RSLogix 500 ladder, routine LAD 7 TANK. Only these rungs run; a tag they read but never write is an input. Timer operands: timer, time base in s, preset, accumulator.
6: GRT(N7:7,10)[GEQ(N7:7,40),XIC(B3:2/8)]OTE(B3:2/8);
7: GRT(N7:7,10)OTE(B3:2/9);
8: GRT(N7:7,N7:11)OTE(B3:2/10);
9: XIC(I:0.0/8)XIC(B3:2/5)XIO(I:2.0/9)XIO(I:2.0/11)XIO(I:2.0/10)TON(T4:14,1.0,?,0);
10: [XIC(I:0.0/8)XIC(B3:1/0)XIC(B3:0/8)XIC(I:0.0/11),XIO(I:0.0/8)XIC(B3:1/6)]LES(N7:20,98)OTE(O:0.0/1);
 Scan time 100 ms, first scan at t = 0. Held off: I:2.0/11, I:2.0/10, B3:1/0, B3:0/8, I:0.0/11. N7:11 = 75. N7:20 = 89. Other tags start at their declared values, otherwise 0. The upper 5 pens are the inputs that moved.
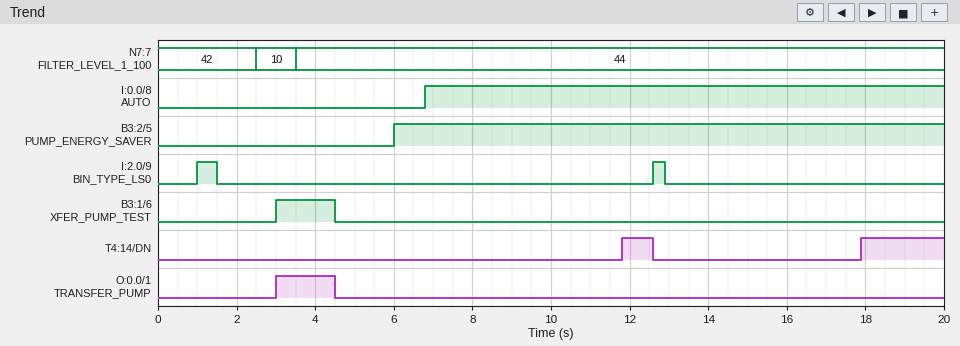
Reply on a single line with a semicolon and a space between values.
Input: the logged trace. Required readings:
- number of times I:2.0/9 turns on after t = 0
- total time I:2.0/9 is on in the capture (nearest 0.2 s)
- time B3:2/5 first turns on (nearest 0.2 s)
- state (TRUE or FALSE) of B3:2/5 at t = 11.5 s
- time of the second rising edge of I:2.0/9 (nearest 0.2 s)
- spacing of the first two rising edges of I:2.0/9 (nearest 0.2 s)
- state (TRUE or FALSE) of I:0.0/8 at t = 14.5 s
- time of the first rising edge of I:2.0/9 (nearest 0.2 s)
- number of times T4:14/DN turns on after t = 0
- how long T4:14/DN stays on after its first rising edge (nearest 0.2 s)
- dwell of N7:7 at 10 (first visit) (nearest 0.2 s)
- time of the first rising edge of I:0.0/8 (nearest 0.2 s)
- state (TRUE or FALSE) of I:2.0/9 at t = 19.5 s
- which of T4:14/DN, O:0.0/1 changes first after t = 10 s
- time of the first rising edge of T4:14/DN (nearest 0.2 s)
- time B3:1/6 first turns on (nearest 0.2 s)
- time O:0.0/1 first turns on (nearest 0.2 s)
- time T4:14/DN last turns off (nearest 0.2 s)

2; 0.8 s; 6.0 s; TRUE; 12.6 s; 11.6 s; TRUE; 1.0 s; 2; 0.8 s; 1.0 s; 6.8 s; FALSE; T4:14/DN; 11.8 s; 3.0 s; 3.0 s; 12.6 s
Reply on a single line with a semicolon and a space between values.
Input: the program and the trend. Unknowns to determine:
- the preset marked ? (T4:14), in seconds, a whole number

5 s
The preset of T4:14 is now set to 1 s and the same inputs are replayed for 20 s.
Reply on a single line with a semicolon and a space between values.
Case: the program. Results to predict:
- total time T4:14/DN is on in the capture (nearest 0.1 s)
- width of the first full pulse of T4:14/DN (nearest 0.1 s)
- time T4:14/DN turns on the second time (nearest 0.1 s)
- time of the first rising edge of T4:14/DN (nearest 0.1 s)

10.9 s; 4.8 s; 13.9 s; 7.8 s
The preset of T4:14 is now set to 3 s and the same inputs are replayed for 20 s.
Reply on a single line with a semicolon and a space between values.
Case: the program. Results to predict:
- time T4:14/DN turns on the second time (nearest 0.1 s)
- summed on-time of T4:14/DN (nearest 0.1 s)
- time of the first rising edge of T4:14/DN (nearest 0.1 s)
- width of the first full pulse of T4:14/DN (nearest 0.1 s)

15.9 s; 6.9 s; 9.8 s; 2.8 s
